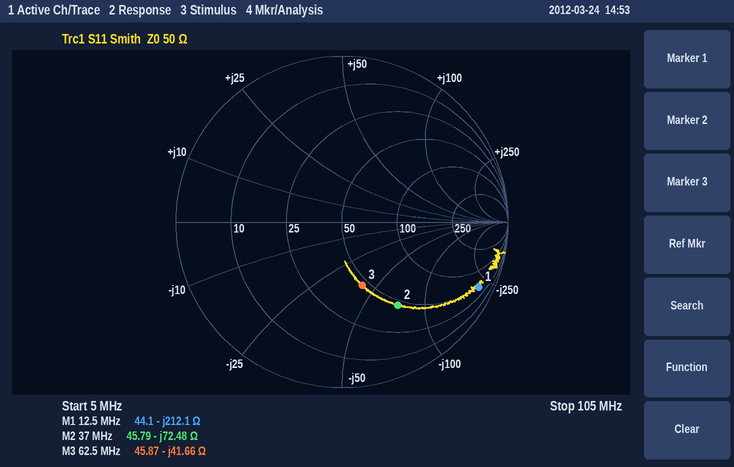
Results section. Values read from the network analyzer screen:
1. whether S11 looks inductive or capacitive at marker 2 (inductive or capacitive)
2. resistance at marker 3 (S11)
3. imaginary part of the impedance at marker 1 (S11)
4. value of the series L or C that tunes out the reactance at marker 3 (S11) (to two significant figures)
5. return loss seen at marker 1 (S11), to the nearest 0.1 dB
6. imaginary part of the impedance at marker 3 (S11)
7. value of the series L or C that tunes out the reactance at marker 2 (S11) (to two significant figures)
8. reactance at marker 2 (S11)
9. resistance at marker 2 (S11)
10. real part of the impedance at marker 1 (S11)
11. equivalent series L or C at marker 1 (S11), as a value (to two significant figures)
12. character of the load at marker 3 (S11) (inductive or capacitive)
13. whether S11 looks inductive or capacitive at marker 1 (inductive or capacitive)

capacitive
45.87 Ω
-212.1 Ω
110 nH
0.8 dB
-41.66 Ω
310 nH
-72.48 Ω
45.79 Ω
44.1 Ω
60 pF
capacitive
capacitive
